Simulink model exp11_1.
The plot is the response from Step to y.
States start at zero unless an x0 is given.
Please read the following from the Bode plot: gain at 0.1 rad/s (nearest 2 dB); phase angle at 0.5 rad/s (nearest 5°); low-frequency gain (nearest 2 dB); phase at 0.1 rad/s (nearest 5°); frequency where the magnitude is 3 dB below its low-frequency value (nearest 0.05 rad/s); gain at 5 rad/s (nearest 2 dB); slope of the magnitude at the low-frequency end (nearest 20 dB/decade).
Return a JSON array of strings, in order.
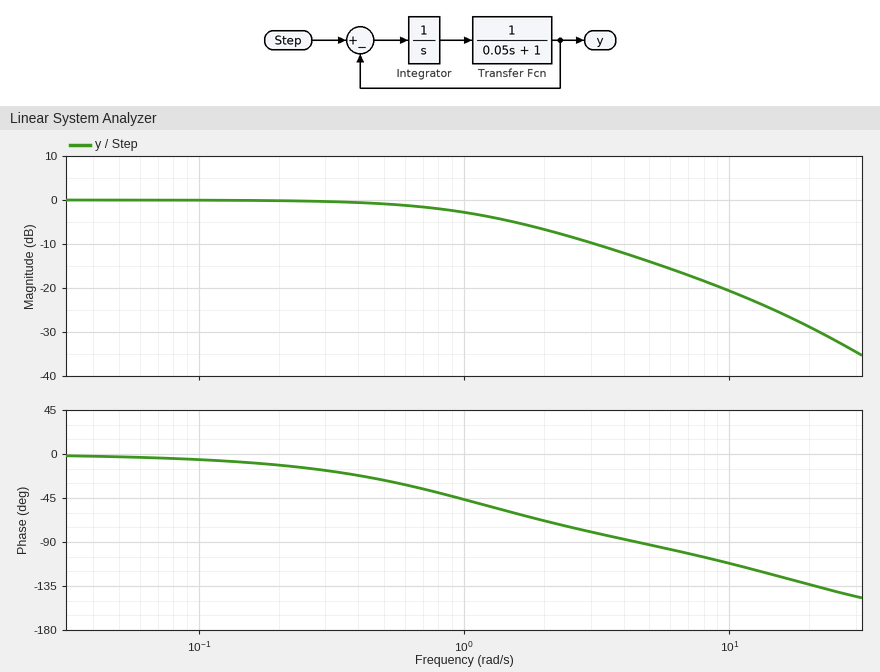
["0 dB", "-25°", "0 dB", "-5°", "1.05 rad/s", "-14 dB", "0 dB/decade"]
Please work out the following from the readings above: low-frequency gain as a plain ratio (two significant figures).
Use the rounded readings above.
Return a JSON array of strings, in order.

["1.0"]
